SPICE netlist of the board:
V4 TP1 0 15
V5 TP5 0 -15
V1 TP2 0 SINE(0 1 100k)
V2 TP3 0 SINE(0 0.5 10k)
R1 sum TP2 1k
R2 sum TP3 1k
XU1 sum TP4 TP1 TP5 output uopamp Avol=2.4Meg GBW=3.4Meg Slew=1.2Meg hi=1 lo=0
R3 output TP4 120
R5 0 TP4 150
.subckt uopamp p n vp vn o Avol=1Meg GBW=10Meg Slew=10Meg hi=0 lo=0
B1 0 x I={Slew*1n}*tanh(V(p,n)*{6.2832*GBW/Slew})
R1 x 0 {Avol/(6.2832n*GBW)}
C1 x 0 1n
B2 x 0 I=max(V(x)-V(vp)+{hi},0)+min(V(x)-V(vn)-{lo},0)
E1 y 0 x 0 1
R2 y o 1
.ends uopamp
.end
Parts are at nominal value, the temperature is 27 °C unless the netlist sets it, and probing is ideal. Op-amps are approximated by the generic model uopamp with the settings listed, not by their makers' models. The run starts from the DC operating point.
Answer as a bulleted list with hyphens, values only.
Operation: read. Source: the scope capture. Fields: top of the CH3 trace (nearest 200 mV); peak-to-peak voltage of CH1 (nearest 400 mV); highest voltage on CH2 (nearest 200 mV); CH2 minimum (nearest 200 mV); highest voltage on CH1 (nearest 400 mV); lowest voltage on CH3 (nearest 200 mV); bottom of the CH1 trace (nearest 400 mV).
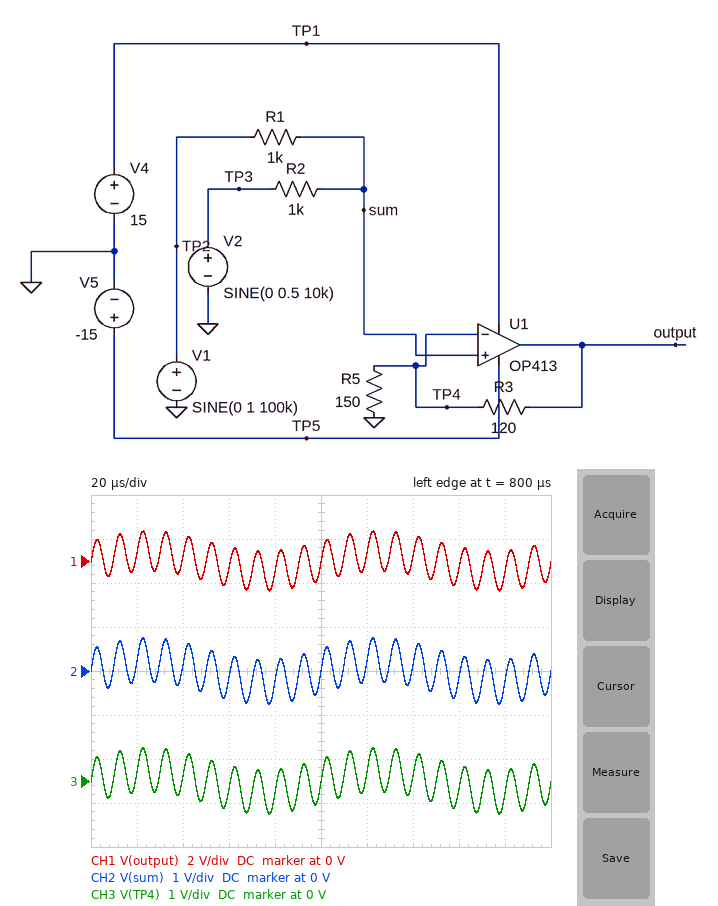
- 800 mV
- 2.8 V
- 800 mV
- -800 mV
- 1.2 V
- -800 mV
- -1.2 V
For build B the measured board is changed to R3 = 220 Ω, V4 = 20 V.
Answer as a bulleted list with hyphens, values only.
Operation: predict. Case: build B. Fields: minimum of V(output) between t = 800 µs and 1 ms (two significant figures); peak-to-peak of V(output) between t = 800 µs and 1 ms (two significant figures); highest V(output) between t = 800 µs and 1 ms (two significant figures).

- -1.8 V
- 3.7 V
- 1.8 V
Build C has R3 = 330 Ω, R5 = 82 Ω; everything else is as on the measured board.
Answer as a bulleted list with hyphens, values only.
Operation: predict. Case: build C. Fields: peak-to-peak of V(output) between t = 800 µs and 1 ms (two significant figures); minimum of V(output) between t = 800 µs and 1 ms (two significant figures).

- 7.3 V
- -3.7 V
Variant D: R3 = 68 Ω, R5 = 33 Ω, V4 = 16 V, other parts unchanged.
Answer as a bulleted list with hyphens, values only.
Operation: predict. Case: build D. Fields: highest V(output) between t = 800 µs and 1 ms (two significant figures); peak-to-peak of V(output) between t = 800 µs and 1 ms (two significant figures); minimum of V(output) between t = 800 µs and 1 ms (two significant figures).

- 2.3 V
- 4.6 V
- -2.3 V
